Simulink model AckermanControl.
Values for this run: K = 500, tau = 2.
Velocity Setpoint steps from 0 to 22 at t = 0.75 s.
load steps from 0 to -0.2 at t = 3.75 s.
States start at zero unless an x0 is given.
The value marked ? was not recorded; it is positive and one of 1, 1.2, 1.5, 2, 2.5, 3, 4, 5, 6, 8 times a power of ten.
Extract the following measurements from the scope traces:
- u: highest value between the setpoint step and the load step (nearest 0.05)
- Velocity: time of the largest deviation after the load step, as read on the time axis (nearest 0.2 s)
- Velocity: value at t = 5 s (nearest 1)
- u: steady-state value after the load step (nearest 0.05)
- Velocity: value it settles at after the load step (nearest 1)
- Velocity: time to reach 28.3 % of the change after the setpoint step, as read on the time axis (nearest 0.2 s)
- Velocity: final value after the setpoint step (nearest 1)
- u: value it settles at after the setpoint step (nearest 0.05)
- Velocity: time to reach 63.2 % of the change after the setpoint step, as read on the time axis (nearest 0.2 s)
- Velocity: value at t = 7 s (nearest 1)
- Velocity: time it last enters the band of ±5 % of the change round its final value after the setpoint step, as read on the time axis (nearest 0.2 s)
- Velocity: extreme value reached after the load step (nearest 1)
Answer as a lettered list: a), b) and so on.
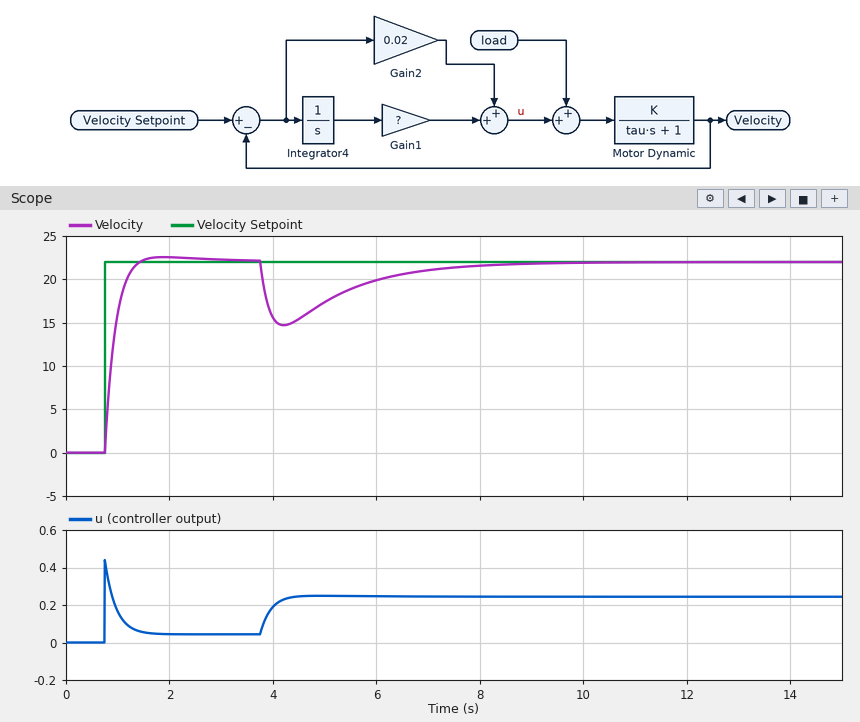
a) 0.45
b) 4.2 s
c) 17
d) 0.25
e) 22
f) 0.8 s
g) 22
h) 0.05
i) 1.0 s
j) 21
k) 1.2 s
l) 15
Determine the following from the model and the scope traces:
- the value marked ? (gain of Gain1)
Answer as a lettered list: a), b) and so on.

a) 0.015
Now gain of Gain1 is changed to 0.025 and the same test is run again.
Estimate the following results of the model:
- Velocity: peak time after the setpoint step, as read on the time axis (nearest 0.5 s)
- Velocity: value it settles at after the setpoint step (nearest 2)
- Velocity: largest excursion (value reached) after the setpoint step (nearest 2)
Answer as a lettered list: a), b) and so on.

a) 1.5 s
b) 22
c) 24
